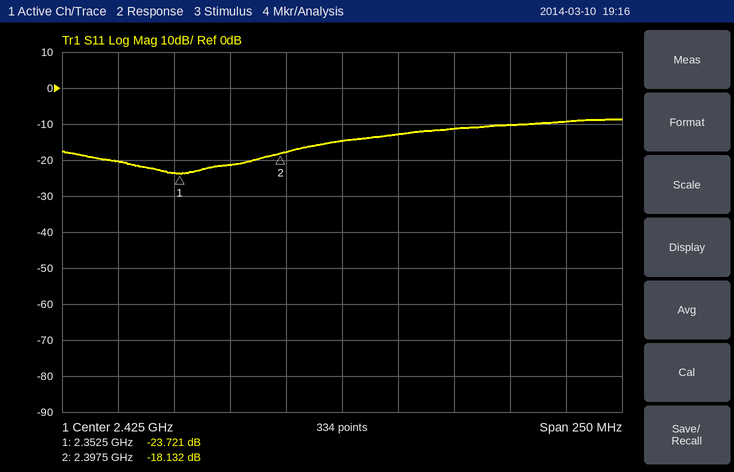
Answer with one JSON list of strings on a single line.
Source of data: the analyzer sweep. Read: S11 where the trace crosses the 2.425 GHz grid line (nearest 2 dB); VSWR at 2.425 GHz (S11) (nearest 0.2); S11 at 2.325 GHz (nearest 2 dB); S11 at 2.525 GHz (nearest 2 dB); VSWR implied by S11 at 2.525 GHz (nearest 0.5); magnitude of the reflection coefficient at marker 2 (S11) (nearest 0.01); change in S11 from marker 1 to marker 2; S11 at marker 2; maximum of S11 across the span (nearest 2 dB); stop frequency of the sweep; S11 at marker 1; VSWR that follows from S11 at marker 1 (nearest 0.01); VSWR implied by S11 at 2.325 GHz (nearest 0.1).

["-14 dB", "1.4", "-20 dB", "-10 dB", "2.0", "0.12", "5.589 dB", "-18.132 dB", "-8 dB", "2.55 GHz", "-23.721 dB", "1.14", "1.2"]
